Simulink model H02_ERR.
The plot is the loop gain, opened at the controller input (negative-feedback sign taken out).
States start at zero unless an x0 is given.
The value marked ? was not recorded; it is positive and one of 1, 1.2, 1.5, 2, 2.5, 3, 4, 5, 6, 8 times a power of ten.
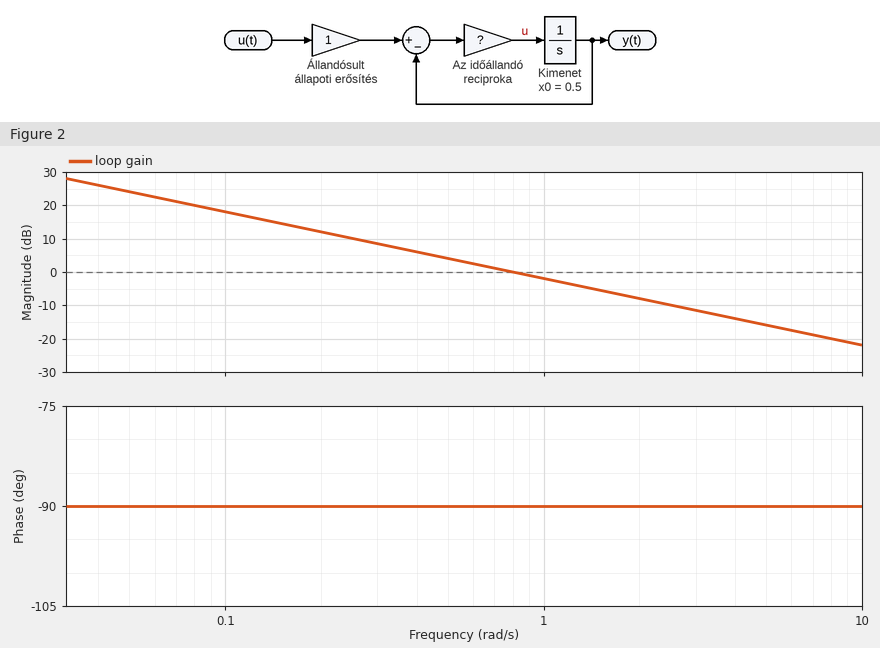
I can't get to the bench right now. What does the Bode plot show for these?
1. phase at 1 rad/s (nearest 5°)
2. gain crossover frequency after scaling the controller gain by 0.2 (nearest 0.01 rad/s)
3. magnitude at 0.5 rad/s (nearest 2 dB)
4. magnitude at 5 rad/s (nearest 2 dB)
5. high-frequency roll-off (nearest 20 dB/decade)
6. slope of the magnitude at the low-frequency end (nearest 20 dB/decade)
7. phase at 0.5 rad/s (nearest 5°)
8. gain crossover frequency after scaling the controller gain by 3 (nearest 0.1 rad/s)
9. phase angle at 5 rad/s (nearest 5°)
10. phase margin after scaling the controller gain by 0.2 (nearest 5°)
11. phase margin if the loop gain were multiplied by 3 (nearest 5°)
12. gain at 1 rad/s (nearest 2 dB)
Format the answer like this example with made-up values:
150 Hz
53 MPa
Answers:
-90°
0.16 rad/s
4 dB
-16 dB
-20 dB/decade
-20 dB/decade
-90°
2.4 rad/s
-90°
90°
90°
-2 dB
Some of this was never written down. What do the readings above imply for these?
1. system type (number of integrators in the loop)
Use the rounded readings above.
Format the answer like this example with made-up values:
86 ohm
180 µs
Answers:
1
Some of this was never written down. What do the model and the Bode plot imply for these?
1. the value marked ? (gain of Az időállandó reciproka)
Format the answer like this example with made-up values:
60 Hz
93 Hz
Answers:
0.8
